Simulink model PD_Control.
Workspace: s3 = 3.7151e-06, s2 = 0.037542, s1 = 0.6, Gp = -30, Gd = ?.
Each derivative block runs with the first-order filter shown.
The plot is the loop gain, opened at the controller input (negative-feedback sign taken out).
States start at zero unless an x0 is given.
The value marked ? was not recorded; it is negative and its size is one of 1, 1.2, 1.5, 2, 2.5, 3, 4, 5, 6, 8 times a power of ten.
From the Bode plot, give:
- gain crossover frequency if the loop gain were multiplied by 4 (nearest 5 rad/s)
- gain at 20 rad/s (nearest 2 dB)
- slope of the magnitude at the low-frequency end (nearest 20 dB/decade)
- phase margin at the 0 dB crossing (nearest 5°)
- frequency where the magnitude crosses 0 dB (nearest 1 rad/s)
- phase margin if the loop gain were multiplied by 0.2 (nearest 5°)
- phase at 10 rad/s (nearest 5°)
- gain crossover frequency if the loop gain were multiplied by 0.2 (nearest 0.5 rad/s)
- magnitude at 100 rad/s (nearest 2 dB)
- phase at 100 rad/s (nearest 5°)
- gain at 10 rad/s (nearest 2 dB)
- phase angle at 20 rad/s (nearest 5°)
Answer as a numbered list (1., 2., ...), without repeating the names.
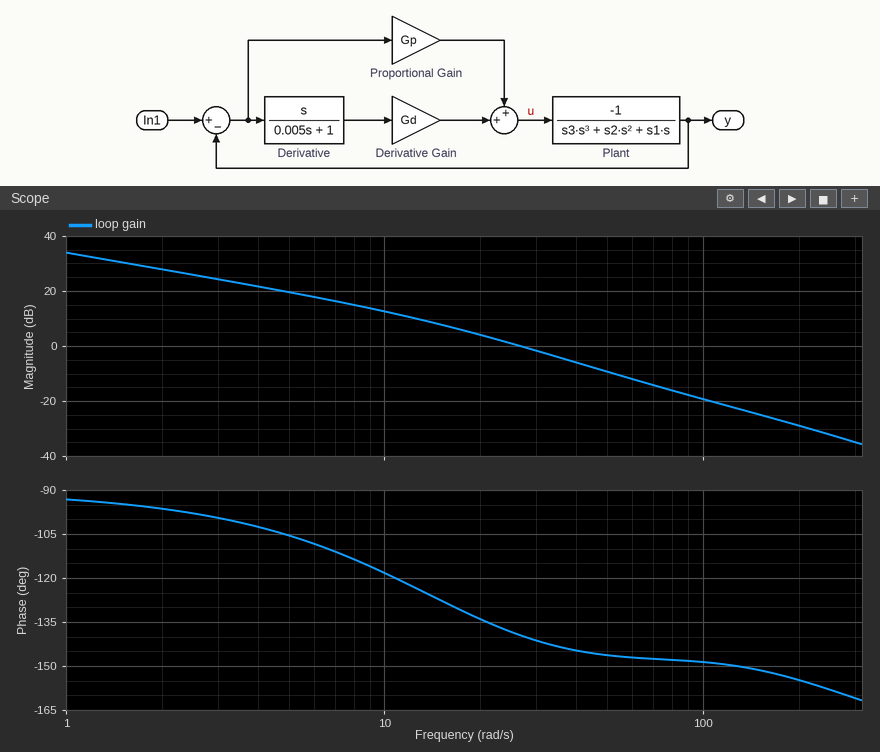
1. 60 rad/s
2. 4 dB
3. -20 dB/decade
4. 40°
5. 27 rad/s
6. 65°
7. -120°
8. 9.0 rad/s
9. -20 dB
10. -150°
11. 12 dB
12. -135°
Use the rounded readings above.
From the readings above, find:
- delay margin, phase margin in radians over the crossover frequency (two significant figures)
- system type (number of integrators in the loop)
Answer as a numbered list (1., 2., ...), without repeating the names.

1. 0.026 s
2. 1
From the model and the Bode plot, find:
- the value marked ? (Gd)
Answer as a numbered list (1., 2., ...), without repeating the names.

1. -0.2
